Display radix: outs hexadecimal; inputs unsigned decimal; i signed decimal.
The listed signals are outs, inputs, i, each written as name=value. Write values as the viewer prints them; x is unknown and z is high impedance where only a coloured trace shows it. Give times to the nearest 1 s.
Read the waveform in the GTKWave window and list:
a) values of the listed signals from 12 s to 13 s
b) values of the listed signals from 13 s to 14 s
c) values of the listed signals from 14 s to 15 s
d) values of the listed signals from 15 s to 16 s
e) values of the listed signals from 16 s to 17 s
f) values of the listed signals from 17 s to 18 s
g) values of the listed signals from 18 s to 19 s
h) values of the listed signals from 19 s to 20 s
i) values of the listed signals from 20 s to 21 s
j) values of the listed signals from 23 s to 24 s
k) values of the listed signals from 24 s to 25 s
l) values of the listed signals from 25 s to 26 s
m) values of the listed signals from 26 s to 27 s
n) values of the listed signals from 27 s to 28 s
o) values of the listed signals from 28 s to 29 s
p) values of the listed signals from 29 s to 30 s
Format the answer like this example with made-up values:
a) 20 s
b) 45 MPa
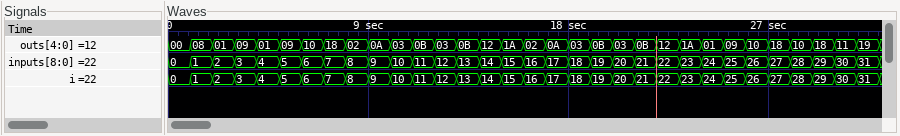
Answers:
a) outs=03, inputs=12, i=12
b) outs=0B, inputs=13, i=13
c) outs=12, inputs=14, i=14
d) outs=1A, inputs=15, i=15
e) outs=02, inputs=16, i=16
f) outs=0A, inputs=17, i=17
g) outs=03, inputs=18, i=18
h) outs=0B, inputs=19, i=19
i) outs=03, inputs=20, i=20
j) outs=1A, inputs=23, i=23
k) outs=01, inputs=24, i=24
l) outs=09, inputs=25, i=25
m) outs=10, inputs=26, i=26
n) outs=18, inputs=27, i=27
o) outs=10, inputs=28, i=28
p) outs=18, inputs=29, i=29
